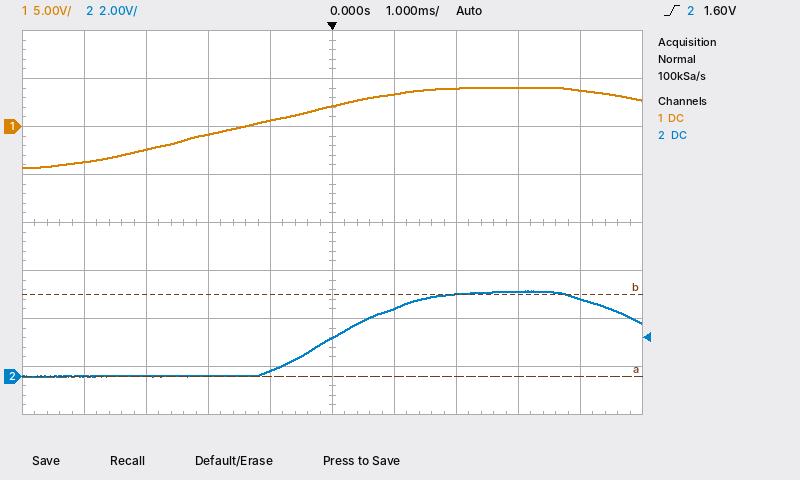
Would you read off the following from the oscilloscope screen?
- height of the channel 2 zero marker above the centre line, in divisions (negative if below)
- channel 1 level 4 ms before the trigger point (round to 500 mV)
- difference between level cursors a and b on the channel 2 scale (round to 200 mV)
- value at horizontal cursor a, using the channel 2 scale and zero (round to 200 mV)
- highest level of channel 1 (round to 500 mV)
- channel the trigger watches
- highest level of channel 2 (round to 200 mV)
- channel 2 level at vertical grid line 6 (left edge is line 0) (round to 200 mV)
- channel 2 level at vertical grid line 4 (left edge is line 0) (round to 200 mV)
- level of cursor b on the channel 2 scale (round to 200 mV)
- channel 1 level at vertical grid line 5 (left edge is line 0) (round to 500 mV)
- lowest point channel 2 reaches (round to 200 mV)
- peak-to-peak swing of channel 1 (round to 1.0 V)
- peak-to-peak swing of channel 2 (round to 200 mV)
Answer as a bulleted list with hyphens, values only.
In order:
- -3.2 div
- -3.5 V
- 3.4 V
- 0.0 V
- 4.0 V
- channel 2
- 3.6 V
- 2.8 V
- 200 mV
- 3.4 V
- 2.0 V
- 0.0 V
- 8.0 V
- 3.6 V
